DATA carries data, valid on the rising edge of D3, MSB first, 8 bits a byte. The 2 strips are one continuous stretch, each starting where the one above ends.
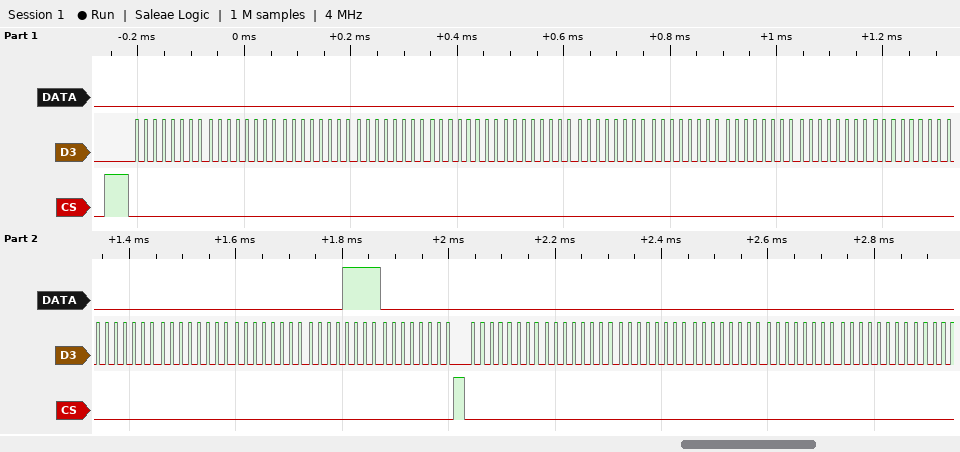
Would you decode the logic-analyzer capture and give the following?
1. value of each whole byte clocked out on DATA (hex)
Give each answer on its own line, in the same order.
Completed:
00 00 00 00 00 00 00 00 00 00 00 00 00 00 0F 00 00 00 00 00 00 00
